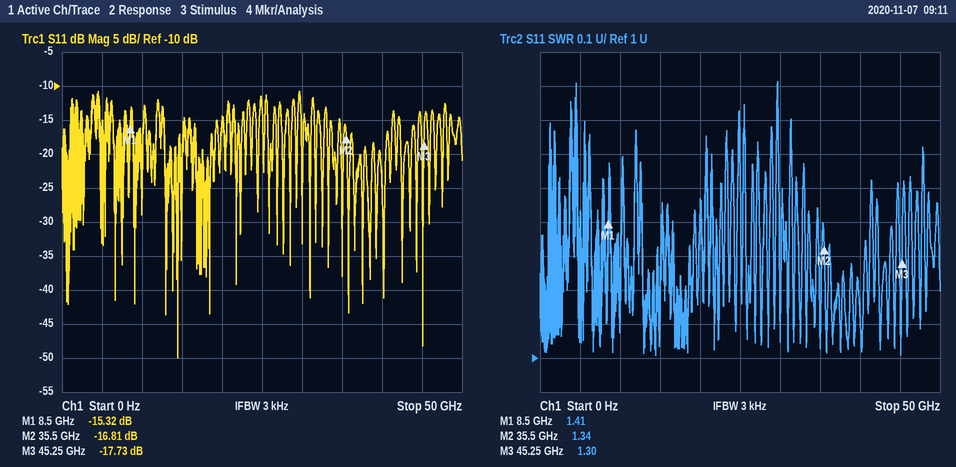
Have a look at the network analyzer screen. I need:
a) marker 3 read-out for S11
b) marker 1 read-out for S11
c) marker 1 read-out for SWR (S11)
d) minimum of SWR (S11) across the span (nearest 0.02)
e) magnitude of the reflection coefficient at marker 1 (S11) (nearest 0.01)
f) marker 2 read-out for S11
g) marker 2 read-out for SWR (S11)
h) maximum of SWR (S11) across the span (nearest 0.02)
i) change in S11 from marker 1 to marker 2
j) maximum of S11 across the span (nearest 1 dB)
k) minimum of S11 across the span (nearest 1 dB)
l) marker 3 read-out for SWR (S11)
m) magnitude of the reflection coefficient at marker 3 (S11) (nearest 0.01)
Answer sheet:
-17.73 dB
-15.32 dB
1.41
1.00
0.17
-16.81 dB
1.34
1.82
-1.49 dB
-11 dB
-50 dB
1.30
0.13
